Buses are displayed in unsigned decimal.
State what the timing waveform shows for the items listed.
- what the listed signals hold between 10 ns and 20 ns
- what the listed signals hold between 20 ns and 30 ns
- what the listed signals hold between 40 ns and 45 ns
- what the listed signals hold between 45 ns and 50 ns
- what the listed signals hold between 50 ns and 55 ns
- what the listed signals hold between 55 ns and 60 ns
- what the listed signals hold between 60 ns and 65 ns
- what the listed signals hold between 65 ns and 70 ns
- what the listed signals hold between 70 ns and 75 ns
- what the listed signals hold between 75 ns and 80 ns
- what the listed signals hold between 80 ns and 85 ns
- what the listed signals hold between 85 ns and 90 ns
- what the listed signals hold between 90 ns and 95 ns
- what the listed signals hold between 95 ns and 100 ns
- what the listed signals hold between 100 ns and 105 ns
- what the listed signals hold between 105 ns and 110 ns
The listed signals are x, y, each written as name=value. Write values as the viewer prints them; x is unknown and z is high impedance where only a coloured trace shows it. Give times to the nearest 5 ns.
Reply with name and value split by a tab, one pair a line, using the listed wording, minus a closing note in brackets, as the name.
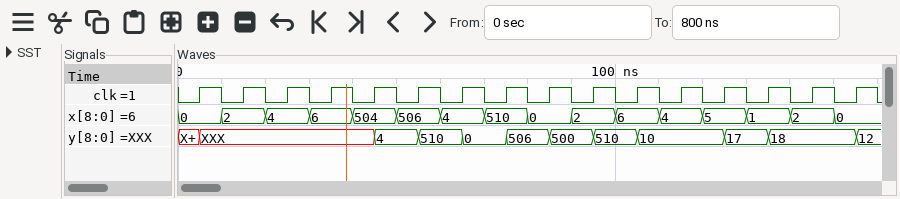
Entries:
what the listed signals hold between 10 ns and 20 ns	x=2, y=XXX
what the listed signals hold between 20 ns and 30 ns	x=4, y=XXX
what the listed signals hold between 40 ns and 45 ns	x=504, y=XXX
what the listed signals hold between 45 ns and 50 ns	x=504, y=4
what the listed signals hold between 50 ns and 55 ns	x=506, y=4
what the listed signals hold between 55 ns and 60 ns	x=506, y=510
what the listed signals hold between 60 ns and 65 ns	x=4, y=510
what the listed signals hold between 65 ns and 70 ns	x=4, y=0
what the listed signals hold between 70 ns and 75 ns	x=510, y=0
what the listed signals hold between 75 ns and 80 ns	x=510, y=506
what the listed signals hold between 80 ns and 85 ns	x=0, y=506
what the listed signals hold between 85 ns and 90 ns	x=0, y=500
what the listed signals hold between 90 ns and 95 ns	x=2, y=500
what the listed signals hold between 95 ns and 100 ns	x=2, y=510
what the listed signals hold between 100 ns and 105 ns	x=6, y=510
what the listed signals hold between 105 ns and 110 ns	x=6, y=10
